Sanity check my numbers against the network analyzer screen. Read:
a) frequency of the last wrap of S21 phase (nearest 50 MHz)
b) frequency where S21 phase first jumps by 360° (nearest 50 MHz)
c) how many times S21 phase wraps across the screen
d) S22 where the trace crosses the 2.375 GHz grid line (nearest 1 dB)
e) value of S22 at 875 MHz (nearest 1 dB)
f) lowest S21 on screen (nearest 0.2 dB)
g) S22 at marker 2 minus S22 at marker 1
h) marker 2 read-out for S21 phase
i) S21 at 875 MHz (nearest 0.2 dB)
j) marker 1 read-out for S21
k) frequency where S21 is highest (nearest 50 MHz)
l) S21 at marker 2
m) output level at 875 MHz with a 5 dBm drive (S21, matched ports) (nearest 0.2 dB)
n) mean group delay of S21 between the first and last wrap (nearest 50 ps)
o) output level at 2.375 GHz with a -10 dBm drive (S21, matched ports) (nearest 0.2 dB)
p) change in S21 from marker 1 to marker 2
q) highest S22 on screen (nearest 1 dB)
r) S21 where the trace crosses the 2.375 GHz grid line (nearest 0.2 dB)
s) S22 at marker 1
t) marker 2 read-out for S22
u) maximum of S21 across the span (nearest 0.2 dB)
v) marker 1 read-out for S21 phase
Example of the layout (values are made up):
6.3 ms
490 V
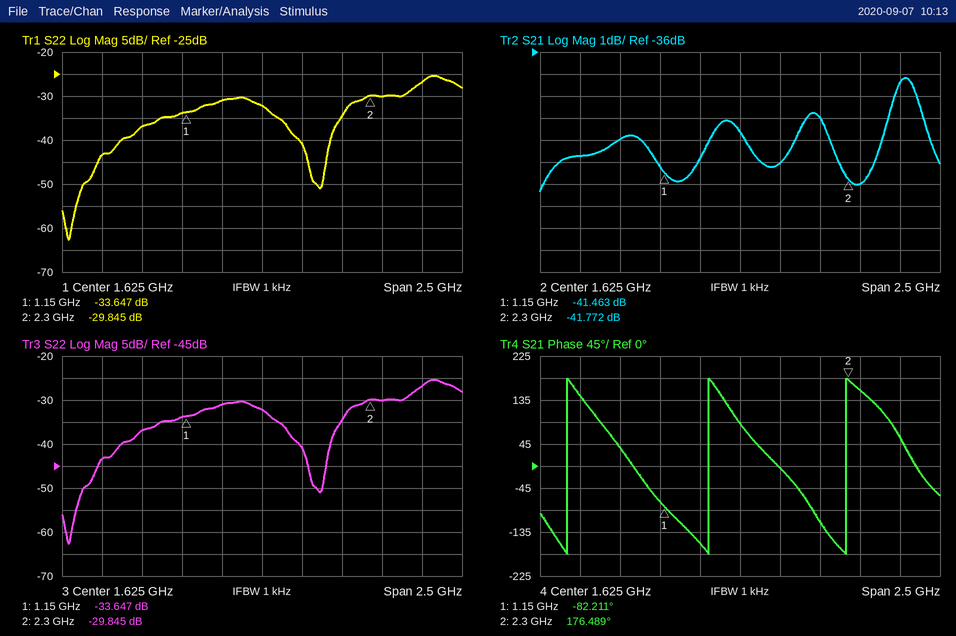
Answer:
2.30 GHz
550 MHz
3
-30 dB
-37 dB
-42.4 dB
3.802 dB
176.489°
-40.0 dB
-41.463 dB
2.65 GHz
-41.772 dB
-35.0 dBm
1.15 ns
-52.0 dBm
-0.309 dB
-25 dB
-42.0 dB
-33.647 dB
-29.845 dB
-37.2 dB
-82.211°
